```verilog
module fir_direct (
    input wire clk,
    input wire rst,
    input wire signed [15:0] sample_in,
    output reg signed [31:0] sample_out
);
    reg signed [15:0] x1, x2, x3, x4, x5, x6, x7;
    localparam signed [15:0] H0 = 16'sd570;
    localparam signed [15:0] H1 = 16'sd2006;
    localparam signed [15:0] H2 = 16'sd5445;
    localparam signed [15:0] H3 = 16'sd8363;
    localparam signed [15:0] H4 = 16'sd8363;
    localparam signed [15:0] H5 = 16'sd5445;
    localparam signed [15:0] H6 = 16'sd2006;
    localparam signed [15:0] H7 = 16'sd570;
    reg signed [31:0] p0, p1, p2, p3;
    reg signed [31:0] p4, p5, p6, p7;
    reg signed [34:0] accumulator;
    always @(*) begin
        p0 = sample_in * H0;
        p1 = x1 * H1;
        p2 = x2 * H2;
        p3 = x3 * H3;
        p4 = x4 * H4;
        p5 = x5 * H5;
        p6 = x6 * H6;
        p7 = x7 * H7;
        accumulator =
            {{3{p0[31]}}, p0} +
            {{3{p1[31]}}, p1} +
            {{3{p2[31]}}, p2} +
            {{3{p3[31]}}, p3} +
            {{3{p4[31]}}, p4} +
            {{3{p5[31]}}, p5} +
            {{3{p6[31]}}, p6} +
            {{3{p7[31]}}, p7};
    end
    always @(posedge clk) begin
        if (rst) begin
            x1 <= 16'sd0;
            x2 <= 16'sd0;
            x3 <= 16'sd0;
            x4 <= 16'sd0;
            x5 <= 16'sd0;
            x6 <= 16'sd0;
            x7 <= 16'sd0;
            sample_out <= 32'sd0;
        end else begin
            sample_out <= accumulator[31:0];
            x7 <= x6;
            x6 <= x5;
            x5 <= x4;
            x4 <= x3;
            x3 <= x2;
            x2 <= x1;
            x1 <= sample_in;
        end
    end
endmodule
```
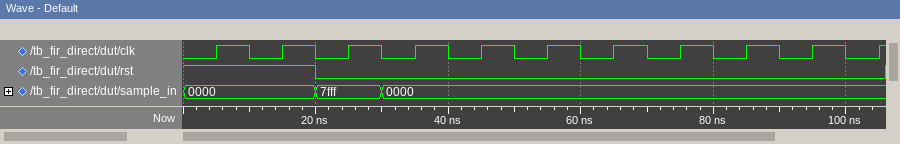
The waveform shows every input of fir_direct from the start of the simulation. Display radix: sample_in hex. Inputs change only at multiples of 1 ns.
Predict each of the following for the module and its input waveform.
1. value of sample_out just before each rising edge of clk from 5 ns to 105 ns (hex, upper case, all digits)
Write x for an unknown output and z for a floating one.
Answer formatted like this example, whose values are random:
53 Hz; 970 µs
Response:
x, 00000000, 00000000, 011CFDC6, 03EAF82A, 0AA26ABB, 10555F55, 10555F55, 0AA26ABB, 03EAF82A, 011CFDC6
